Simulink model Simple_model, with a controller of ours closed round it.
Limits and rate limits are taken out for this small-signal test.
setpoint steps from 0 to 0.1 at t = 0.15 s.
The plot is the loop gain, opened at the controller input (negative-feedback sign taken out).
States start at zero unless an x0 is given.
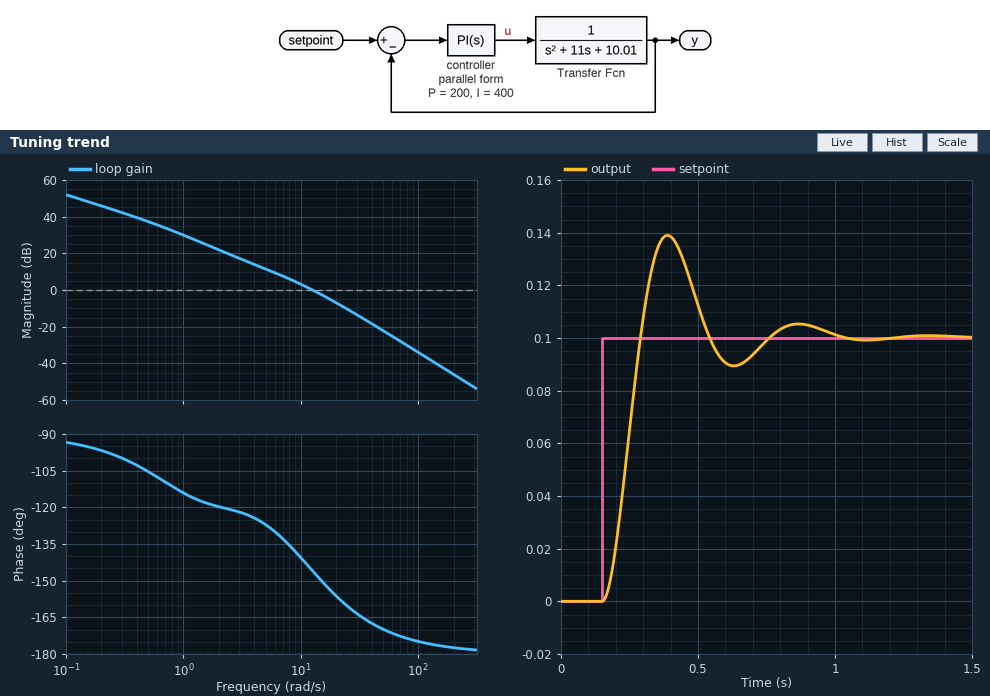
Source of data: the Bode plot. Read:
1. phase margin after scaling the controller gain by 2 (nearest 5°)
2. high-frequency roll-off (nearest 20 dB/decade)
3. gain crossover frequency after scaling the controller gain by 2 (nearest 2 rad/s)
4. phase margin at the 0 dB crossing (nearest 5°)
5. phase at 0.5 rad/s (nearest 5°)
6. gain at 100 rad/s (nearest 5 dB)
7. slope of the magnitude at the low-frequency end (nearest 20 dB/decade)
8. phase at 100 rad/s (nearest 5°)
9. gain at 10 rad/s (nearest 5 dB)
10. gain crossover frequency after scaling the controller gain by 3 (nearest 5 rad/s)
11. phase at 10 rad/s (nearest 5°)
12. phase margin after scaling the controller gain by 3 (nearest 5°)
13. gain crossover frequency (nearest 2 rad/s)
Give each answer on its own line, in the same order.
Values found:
25°
-40 dB/decade
18 rad/s
35°
-105°
-35 dB
-20 dB/decade
-175°
5 dB
25 rad/s
-140°
20°
12 rad/s
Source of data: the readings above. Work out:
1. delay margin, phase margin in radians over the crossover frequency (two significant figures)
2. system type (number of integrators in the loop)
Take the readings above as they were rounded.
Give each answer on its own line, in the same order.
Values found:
0.051 s
1
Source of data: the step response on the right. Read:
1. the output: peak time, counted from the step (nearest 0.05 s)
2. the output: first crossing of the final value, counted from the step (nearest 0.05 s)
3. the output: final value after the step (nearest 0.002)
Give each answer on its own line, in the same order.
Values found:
0.25 s
0.15 s
0.100
